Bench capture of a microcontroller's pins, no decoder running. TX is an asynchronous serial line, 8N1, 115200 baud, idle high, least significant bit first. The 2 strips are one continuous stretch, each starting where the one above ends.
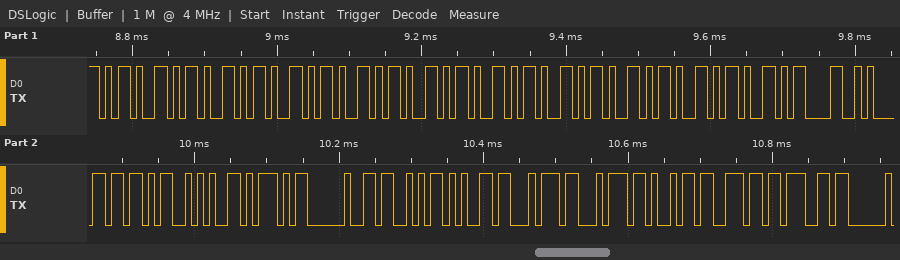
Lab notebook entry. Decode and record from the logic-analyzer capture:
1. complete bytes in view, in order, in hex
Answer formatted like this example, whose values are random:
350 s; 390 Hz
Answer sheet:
0x2D 0x2D 0x2D 0x2D 0x2D 0x2D 0x2D 0x2D 0x2D 0x2D 0x0D 0x0A 0x5B 0x2A 0x5D 0x20 0x53 0x65 0x74 0x74 0x69 0x6E 0x67
